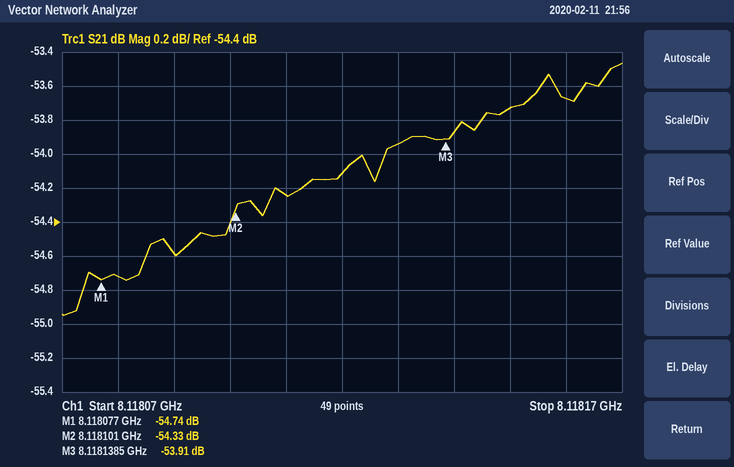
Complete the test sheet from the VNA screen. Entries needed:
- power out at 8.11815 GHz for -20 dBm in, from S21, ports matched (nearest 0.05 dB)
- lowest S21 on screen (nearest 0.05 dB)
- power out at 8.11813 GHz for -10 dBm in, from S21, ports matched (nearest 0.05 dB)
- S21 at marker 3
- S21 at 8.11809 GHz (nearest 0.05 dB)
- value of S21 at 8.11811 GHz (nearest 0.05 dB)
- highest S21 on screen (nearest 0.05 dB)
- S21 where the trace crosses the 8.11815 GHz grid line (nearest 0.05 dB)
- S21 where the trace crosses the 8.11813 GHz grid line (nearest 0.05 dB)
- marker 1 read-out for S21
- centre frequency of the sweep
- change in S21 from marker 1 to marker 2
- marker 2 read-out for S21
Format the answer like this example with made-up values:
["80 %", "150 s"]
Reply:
["-73.75 dBm", "-54.95 dB", "-63.95 dBm", "-53.91 dB", "-54.60 dB", "-54.25 dB", "-53.45 dB", "-53.75 dB", "-53.95 dB", "-54.74 dB", "8.11812 GHz", "0.41 dB", "-54.33 dB"]
